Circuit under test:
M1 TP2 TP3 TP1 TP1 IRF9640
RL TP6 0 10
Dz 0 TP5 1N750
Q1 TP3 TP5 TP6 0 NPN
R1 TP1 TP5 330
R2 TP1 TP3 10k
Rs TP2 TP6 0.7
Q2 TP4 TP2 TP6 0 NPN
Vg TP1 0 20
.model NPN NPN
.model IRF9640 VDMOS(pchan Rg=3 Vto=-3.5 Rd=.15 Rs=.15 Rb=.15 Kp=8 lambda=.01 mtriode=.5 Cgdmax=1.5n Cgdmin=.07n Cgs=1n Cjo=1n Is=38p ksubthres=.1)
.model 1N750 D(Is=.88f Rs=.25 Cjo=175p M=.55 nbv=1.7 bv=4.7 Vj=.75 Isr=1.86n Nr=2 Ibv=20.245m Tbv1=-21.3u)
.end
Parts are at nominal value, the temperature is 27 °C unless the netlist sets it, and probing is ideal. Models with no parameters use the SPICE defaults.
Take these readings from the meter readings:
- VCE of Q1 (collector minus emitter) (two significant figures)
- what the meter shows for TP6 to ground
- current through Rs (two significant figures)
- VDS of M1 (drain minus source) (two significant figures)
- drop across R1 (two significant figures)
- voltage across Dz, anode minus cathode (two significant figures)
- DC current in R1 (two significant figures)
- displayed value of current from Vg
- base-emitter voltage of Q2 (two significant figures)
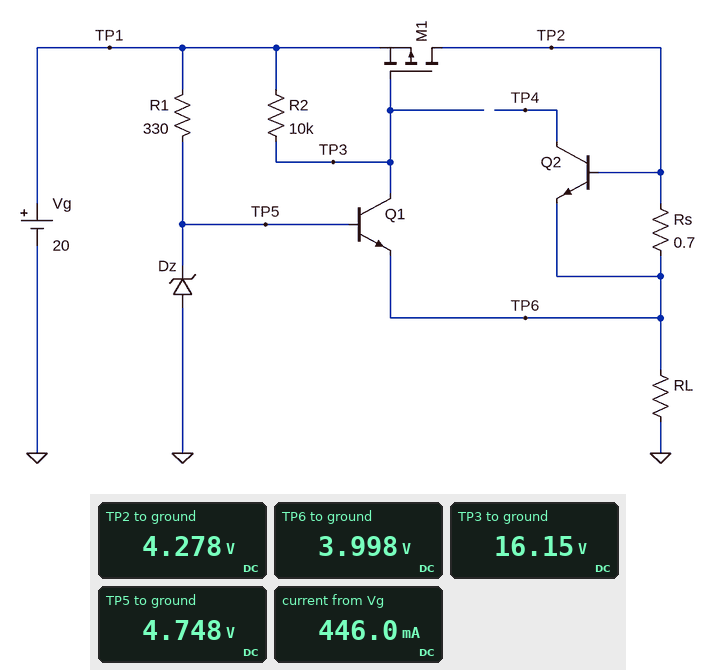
12 V
3.998 V
400 mA
-16 V
15 V
-4.7 V
46 mA
446.0 mA
280 mV
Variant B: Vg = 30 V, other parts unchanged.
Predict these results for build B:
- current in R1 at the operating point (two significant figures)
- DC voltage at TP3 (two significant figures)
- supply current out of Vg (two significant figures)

76 mA
26 V
480 mA
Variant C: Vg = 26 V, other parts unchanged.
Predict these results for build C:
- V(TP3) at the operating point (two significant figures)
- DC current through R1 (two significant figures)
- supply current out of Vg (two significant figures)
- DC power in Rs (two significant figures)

22 V
64 mA
470 mA
110 mW
